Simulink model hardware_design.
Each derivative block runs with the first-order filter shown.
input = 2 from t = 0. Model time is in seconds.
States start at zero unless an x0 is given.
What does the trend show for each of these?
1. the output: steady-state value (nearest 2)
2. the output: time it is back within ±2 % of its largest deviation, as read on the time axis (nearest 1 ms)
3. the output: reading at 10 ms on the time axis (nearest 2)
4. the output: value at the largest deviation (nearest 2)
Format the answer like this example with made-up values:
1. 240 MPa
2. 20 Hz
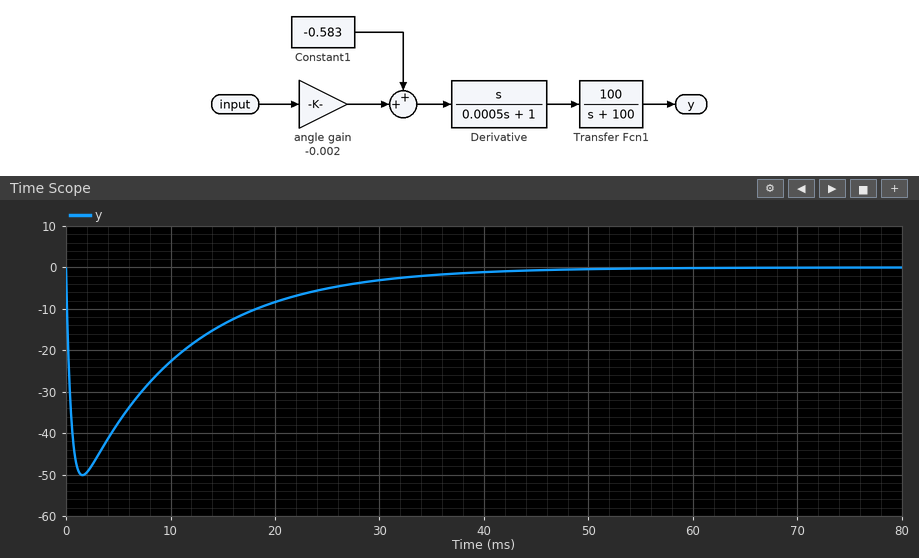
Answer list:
1. 0
2. 41 ms
3. -22
4. -50
